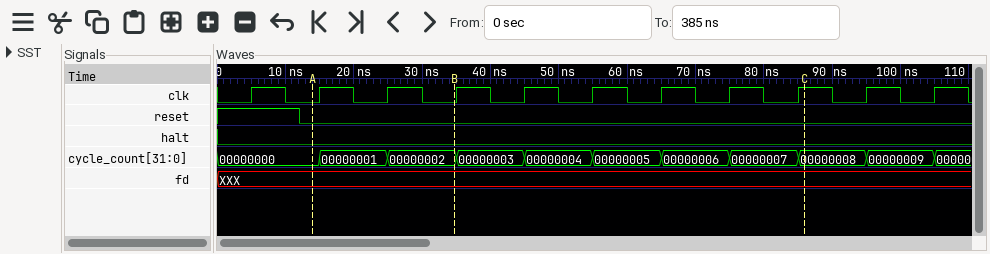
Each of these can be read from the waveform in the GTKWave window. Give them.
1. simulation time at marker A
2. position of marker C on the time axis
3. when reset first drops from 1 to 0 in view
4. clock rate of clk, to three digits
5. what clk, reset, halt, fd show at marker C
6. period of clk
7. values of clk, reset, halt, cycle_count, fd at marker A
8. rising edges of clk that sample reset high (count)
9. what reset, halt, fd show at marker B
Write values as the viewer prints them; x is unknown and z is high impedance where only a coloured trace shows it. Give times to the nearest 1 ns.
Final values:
14 ns
86 ns
12 ns
100 MHz
clk=1, reset=0, halt=0, fd=XXX
10 ns
clk=0, reset=0, halt=0, cycle_count=00000000, fd=XXX
1
reset=0, halt=0, fd=XXX
